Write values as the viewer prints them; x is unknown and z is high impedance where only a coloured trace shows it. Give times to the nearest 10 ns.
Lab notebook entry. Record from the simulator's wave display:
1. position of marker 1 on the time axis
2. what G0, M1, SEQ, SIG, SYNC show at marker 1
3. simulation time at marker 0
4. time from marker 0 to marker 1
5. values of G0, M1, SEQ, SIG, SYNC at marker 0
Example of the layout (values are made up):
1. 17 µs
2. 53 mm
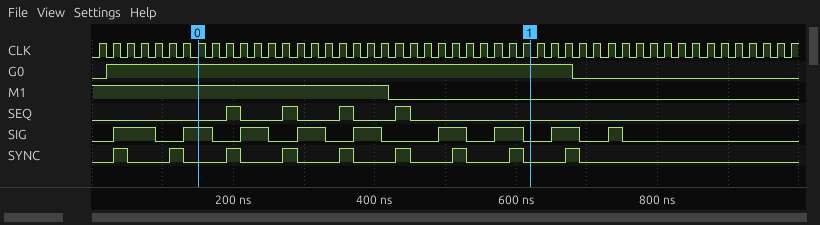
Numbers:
1. 620 ns
2. G0=1, M1=0, SEQ=0, SIG=0, SYNC=0
3. 150 ns
4. 470 ns
5. G0=1, M1=1, SEQ=0, SIG=1, SYNC=0
